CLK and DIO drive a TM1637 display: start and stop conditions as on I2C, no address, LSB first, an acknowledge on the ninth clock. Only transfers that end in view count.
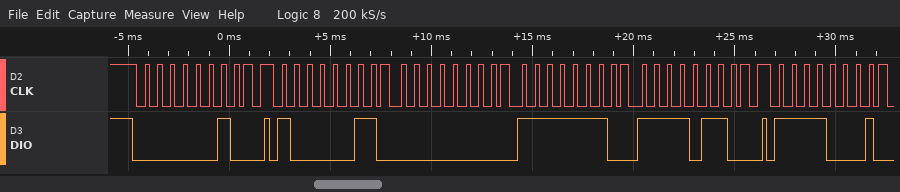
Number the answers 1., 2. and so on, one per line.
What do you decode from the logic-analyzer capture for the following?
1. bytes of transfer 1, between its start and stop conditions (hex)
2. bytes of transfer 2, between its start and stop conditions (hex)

1. 40
2. C1 00 7F 6F
